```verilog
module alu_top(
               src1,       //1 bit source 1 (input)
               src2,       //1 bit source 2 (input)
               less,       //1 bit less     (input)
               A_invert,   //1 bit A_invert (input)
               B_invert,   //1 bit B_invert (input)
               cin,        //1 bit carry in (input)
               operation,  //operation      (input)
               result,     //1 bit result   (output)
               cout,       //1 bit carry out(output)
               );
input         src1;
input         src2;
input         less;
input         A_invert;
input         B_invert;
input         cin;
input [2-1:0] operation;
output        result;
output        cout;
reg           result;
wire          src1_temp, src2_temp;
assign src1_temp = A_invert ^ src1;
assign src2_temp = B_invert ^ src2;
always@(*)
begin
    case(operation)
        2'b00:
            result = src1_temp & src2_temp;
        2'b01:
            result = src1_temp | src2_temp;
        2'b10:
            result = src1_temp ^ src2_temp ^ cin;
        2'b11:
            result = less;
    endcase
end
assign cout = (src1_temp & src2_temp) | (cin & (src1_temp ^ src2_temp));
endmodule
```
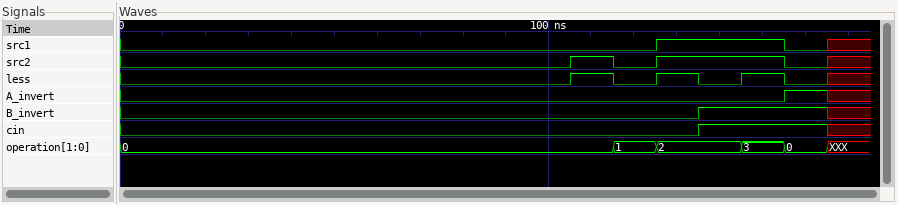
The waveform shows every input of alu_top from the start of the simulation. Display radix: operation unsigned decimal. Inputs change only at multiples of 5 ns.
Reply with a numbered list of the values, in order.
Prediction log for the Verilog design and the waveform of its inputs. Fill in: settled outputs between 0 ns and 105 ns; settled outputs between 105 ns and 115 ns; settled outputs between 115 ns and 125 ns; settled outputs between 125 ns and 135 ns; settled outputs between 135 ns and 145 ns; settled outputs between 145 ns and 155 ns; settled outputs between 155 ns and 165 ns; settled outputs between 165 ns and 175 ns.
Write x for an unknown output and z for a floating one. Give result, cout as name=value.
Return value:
1. result=0, cout=0
2. result=0, cout=0
3. result=0, cout=0
4. result=0, cout=1
5. result=0, cout=1
6. result=1, cout=1
7. result=1, cout=1
8. result=1, cout=x
